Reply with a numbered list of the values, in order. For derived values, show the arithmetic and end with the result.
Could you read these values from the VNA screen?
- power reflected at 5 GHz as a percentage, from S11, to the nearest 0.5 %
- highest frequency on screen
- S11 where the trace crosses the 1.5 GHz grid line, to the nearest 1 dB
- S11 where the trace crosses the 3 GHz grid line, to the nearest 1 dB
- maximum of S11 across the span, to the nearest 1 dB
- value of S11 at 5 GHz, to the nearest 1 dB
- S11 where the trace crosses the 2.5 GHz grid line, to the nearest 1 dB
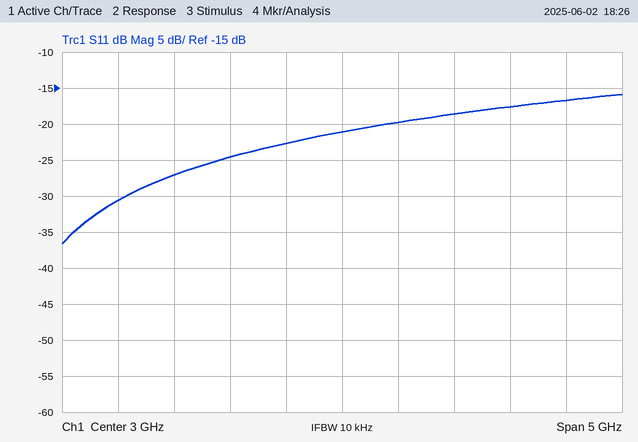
1. 10^(-17/10) ≈ 2.0 %
2. 5.5 GHz
3. -27 dB
4. -21 dB
5. -16 dB
6. -17 dB
7. -23 dB
